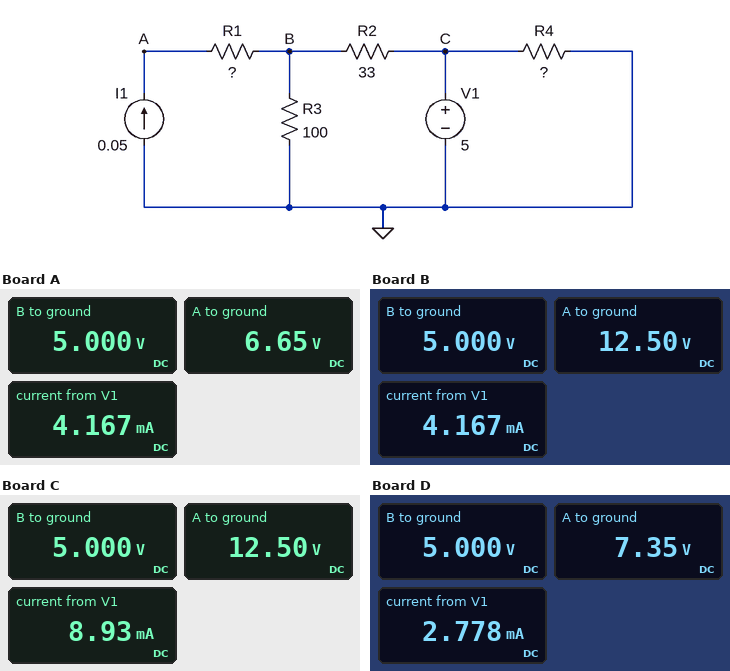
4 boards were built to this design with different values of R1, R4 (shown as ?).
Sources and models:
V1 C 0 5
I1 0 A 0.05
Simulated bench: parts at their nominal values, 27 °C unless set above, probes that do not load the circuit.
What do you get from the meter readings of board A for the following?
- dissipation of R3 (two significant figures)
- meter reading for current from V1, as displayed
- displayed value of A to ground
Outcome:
250 mW
4.167 mA
6.65 V
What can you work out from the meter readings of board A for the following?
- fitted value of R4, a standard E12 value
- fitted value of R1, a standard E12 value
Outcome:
1.2 kΩ
33 Ω
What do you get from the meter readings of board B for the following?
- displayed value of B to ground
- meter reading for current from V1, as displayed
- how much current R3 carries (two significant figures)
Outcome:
5.000 V
4.167 mA
50 mA
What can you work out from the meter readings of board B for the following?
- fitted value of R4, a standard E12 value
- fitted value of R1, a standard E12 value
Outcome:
1.2 kΩ
150 Ω
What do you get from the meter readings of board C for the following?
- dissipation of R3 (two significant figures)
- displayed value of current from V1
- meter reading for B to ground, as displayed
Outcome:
250 mW
8.93 mA
5.000 V
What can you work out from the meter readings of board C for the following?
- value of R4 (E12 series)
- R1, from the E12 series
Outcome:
560 Ω
150 Ω
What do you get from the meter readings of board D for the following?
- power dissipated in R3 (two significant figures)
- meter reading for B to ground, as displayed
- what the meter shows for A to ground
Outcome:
250 mW
5.000 V
7.35 V
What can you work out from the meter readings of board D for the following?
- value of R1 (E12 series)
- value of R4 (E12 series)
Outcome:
47 Ω
1.8 kΩ
